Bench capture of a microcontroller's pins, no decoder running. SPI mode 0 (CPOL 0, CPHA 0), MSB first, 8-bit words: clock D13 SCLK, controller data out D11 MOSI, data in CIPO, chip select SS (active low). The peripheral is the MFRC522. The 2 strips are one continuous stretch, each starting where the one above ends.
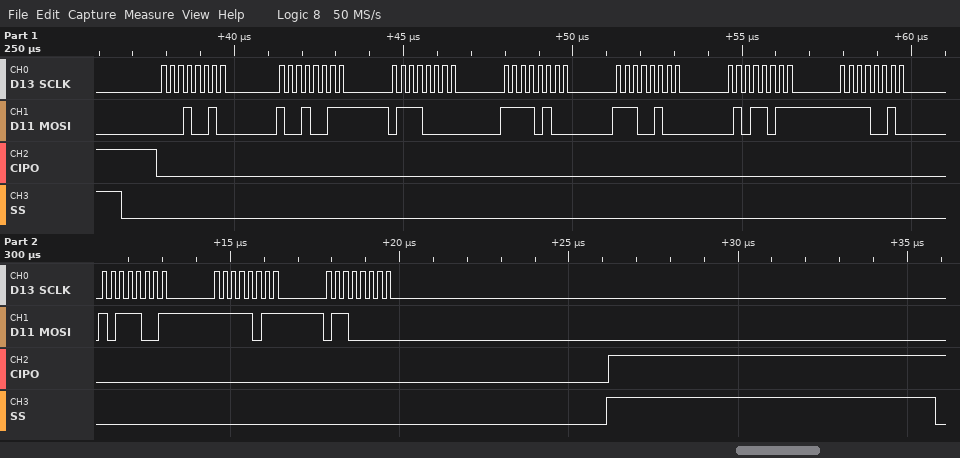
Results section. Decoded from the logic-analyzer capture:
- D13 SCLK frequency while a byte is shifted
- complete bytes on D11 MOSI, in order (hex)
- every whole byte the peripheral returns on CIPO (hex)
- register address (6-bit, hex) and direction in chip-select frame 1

4 MHz
0x12 0x93 0x70 0xF4 0xE4 0x5B 0xF2 0xB9 0xFB 0x60
0x00 0x00 0x00 0x00 0x00 0x00 0x00 0x00 0x00 0x00
0x09 write
